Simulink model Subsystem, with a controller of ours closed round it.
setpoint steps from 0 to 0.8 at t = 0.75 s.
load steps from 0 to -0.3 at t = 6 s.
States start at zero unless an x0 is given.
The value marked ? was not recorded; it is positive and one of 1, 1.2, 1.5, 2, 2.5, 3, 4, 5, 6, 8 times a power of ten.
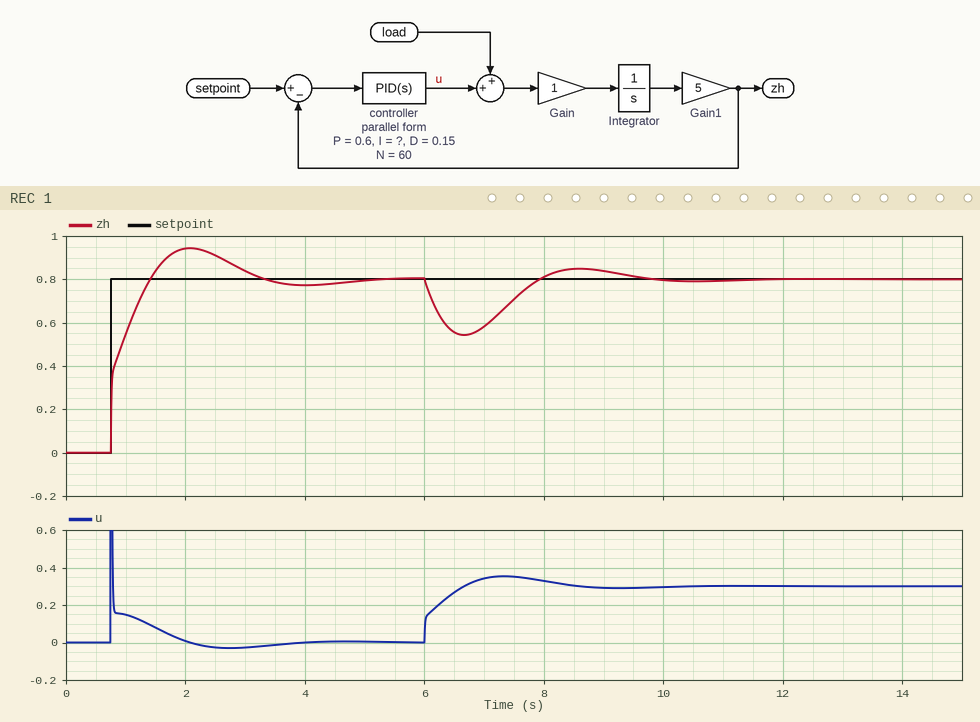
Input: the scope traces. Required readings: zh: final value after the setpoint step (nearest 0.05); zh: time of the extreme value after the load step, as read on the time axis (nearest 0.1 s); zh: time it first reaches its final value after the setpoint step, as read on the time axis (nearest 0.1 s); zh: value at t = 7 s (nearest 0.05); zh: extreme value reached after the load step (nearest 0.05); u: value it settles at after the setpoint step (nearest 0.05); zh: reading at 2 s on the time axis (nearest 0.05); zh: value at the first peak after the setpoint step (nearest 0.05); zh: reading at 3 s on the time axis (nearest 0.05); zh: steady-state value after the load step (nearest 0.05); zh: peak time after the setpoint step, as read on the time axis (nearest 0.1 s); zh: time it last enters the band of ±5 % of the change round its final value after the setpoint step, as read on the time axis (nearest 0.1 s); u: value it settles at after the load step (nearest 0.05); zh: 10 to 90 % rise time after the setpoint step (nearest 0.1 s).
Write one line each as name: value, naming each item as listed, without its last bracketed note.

zh: final value after the setpoint step: 0.80
zh: time of the extreme value after the load step, as read on the time axis: 6.7 s
zh: time it first reaches its final value after the setpoint step, as read on the time axis: 1.4 s
zh: value at t = 7 s: 0.60
zh: extreme value reached after the load step: 0.55
u: value it settles at after the setpoint step: 0.00
zh: reading at 2 s on the time axis: 0.95
zh: value at the first peak after the setpoint step: 0.95
zh: reading at 3 s on the time axis: 0.85
zh: steady-state value after the load step: 0.80
zh: peak time after the setpoint step, as read on the time axis: 2.1 s
zh: time it last enters the band of ±5 % of the change round its final value after the setpoint step, as read on the time axis: 3.0 s
u: value it settles at after the load step: 0.30
zh: 10 to 90 % rise time after the setpoint step: 0.5 s
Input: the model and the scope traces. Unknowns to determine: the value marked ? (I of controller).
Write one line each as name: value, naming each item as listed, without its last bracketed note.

the value marked ?: 1.2
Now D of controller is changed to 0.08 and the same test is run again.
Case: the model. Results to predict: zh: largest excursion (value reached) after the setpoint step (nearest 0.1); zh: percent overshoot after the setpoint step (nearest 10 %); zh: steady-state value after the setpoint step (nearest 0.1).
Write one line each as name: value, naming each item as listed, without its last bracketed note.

zh: largest excursion (value reached) after the setpoint step: 1.0
zh: percent overshoot after the setpoint step: 20 %
zh: steady-state value after the setpoint step: 0.8
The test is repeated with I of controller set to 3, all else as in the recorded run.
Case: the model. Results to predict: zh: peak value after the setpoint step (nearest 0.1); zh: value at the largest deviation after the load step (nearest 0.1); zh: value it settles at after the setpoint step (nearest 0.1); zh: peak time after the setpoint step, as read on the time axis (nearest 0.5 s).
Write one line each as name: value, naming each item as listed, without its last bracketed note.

zh: peak value after the setpoint step: 1.0
zh: value at the largest deviation after the load step: 0.6
zh: value it settles at after the setpoint step: 0.8
zh: peak time after the setpoint step, as read on the time axis: 1.5 s
